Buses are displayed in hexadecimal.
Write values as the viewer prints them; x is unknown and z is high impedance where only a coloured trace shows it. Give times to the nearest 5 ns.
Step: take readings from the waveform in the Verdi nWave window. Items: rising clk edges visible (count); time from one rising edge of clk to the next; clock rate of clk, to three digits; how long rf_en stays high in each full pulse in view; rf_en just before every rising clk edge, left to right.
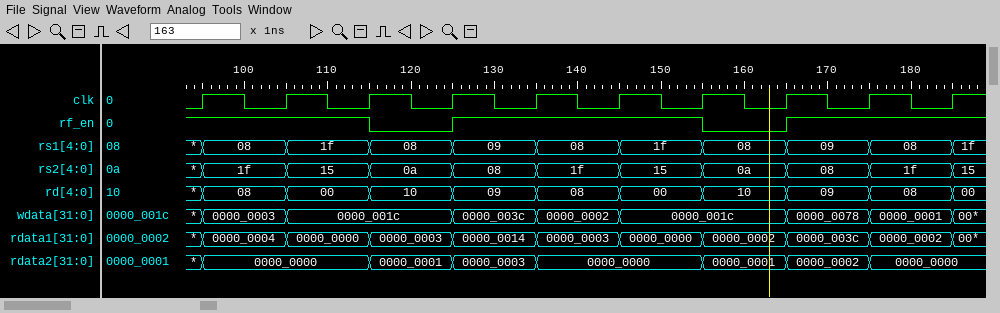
10
10 ns
100 MHz
30 ns
1 1 1 0 1 1 1 0 1 1
